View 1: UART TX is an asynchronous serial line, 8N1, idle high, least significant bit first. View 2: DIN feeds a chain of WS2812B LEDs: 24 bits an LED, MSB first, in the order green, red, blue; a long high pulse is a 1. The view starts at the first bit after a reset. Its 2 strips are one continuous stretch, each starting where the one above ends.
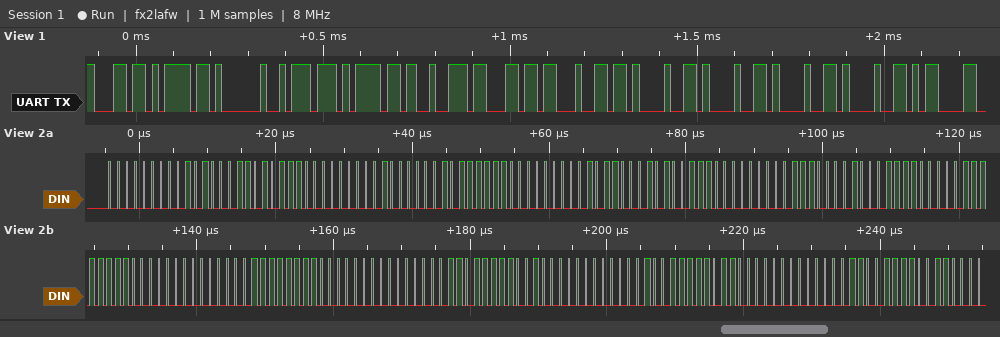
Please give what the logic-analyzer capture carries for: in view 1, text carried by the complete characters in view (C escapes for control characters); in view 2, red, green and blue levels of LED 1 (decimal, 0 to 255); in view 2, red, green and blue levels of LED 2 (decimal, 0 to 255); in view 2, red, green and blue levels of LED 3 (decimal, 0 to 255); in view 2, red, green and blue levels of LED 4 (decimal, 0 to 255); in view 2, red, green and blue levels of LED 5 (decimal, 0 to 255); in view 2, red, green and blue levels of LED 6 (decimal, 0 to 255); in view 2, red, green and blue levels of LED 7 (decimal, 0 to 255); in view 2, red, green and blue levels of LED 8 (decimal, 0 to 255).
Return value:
"lo world!!!!\r"
81, 0, 174
129, 0, 126
177, 0, 78
225, 0, 30
240, 15, 0
192, 63, 0
144, 111, 0
96, 159, 0
